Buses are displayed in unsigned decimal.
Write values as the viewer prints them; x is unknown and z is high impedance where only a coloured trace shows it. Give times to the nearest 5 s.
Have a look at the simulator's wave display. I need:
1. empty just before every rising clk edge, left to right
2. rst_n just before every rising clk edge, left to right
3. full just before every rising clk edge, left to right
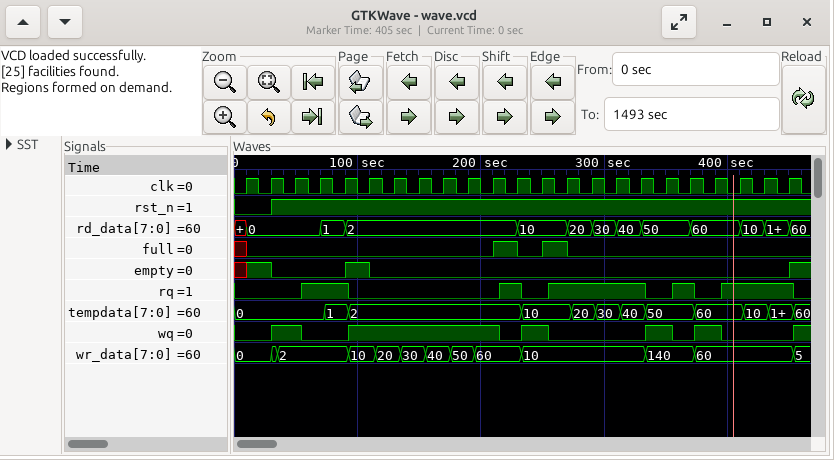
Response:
x 1 0 0 0 1 0 0 0 0 0 0 0 0 0 0 0 0 0 0 0 0 0
0 0 1 1 1 1 1 1 1 1 1 1 1 1 1 1 1 1 1 1 1 1 1
x 0 0 0 0 0 0 0 0 0 0 1 0 1 0 0 0 0 0 0 0 0 0
